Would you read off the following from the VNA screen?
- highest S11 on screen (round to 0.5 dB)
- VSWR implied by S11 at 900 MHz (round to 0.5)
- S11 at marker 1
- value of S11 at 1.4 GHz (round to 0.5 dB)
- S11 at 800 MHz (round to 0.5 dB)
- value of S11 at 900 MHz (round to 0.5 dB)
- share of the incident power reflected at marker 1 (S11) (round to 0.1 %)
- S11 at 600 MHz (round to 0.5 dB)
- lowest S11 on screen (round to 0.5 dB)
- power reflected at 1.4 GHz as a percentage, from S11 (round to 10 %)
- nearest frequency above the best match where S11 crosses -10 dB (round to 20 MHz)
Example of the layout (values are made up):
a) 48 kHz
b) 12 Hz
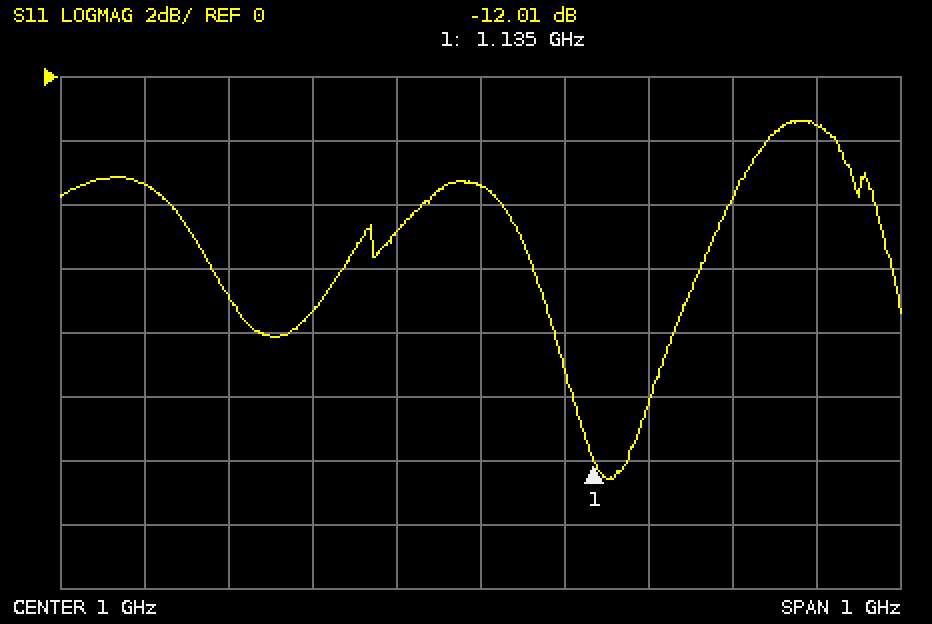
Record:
a) -1.5 dB
b) 3.5
c) -12.01 dB
d) -1.5 dB
e) -7.5 dB
f) -5.0 dB
g) 6.3 %
h) -3.5 dB
i) -12.5 dB
j) 70 %
k) 1.20 GHz
